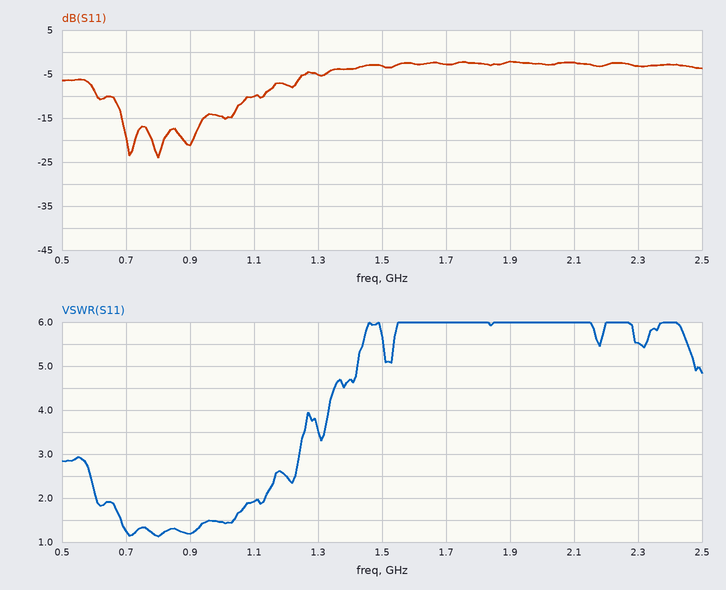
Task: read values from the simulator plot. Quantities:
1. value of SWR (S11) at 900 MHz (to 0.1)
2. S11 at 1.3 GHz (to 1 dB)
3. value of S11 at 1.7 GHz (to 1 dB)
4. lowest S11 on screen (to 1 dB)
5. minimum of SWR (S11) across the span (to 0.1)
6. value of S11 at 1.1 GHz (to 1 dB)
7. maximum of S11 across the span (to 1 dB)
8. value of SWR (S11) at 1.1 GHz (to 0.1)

1.2
-5 dB
-3 dB
-24 dB
1.1
-10 dB
-2 dB
1.9
